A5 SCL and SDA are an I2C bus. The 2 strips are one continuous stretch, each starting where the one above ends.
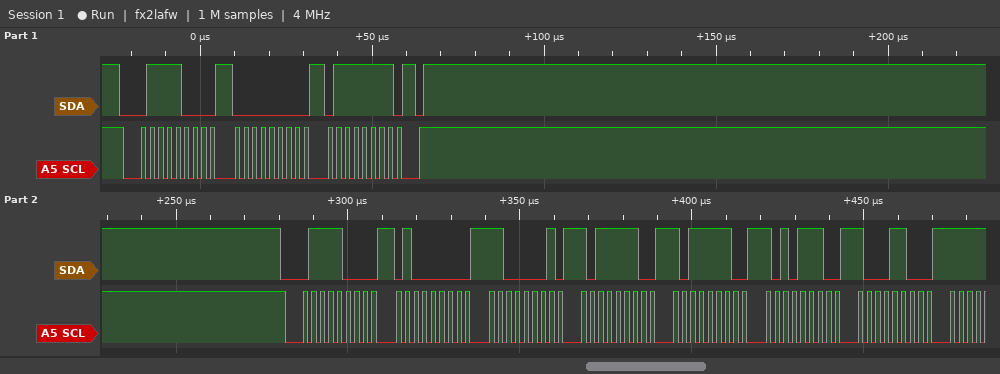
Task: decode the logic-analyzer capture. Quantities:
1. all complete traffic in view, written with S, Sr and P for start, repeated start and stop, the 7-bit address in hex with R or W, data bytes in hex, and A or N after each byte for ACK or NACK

S 3CW A 00 A 7F A P S 3CW A 40 A C1 A BE A BE A AE A 8C A
